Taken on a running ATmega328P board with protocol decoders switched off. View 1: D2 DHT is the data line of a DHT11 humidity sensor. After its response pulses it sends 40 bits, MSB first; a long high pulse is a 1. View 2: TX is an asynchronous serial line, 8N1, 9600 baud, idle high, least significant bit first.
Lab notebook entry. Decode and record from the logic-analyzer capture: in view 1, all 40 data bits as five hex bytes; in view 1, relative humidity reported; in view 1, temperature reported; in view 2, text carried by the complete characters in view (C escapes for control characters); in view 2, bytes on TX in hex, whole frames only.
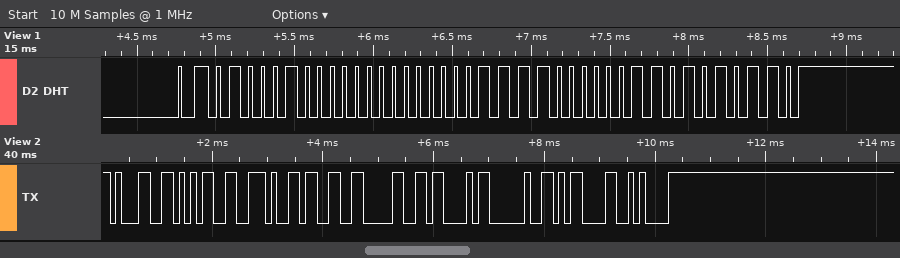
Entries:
44 00 0F 03 56
68 %
15.3 °C
"15.30C \r\n"
0x31 0x35 0x2E 0x33 0x30 0x43 0x20 0x0D 0x0A
